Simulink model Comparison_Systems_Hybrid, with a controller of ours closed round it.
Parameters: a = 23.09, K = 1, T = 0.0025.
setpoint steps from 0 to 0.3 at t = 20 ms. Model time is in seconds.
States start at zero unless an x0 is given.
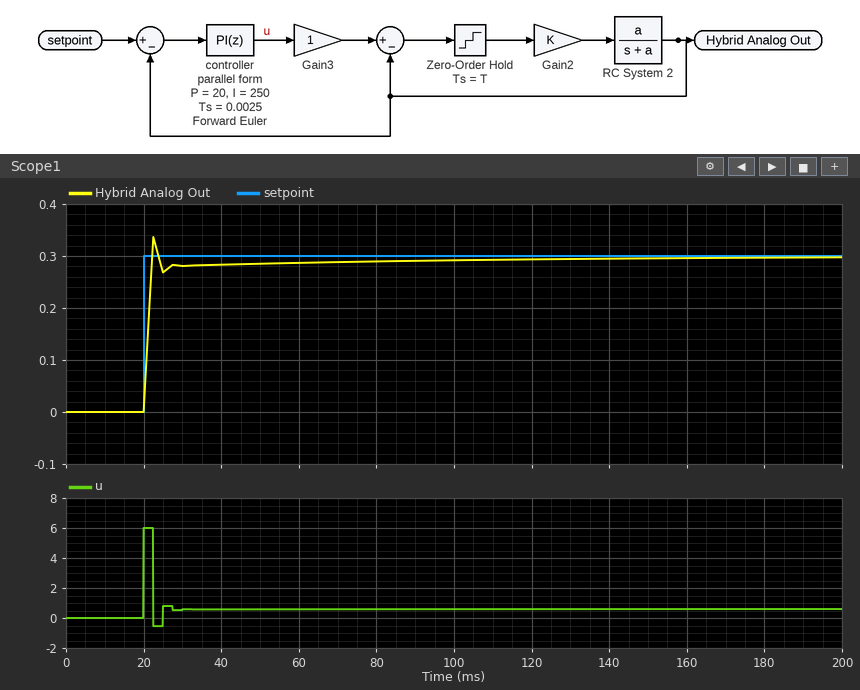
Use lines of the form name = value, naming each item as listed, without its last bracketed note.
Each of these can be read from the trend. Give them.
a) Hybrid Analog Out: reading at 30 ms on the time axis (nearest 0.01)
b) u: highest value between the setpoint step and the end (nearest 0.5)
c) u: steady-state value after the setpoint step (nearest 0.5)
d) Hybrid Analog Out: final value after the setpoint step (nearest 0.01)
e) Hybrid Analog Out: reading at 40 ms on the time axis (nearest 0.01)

Hybrid Analog Out: reading at 30 ms on the time axis = 0.28
u: highest value between the setpoint step and the end = 6.0
u: steady-state value after the setpoint step = 0.5
Hybrid Analog Out: final value after the setpoint step = 0.30
Hybrid Analog Out: reading at 40 ms on the time axis = 0.28
